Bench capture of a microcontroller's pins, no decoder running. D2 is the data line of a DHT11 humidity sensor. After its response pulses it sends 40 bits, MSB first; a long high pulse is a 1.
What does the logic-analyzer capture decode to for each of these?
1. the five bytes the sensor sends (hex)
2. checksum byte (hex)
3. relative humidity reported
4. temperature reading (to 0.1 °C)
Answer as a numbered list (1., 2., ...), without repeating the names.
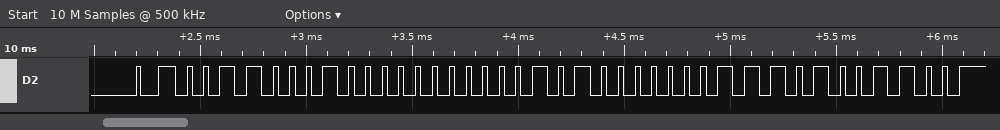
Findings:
1. 31 00 14 07 4C
2. 0x4C
3. 49 %
4. 20.7 °C
